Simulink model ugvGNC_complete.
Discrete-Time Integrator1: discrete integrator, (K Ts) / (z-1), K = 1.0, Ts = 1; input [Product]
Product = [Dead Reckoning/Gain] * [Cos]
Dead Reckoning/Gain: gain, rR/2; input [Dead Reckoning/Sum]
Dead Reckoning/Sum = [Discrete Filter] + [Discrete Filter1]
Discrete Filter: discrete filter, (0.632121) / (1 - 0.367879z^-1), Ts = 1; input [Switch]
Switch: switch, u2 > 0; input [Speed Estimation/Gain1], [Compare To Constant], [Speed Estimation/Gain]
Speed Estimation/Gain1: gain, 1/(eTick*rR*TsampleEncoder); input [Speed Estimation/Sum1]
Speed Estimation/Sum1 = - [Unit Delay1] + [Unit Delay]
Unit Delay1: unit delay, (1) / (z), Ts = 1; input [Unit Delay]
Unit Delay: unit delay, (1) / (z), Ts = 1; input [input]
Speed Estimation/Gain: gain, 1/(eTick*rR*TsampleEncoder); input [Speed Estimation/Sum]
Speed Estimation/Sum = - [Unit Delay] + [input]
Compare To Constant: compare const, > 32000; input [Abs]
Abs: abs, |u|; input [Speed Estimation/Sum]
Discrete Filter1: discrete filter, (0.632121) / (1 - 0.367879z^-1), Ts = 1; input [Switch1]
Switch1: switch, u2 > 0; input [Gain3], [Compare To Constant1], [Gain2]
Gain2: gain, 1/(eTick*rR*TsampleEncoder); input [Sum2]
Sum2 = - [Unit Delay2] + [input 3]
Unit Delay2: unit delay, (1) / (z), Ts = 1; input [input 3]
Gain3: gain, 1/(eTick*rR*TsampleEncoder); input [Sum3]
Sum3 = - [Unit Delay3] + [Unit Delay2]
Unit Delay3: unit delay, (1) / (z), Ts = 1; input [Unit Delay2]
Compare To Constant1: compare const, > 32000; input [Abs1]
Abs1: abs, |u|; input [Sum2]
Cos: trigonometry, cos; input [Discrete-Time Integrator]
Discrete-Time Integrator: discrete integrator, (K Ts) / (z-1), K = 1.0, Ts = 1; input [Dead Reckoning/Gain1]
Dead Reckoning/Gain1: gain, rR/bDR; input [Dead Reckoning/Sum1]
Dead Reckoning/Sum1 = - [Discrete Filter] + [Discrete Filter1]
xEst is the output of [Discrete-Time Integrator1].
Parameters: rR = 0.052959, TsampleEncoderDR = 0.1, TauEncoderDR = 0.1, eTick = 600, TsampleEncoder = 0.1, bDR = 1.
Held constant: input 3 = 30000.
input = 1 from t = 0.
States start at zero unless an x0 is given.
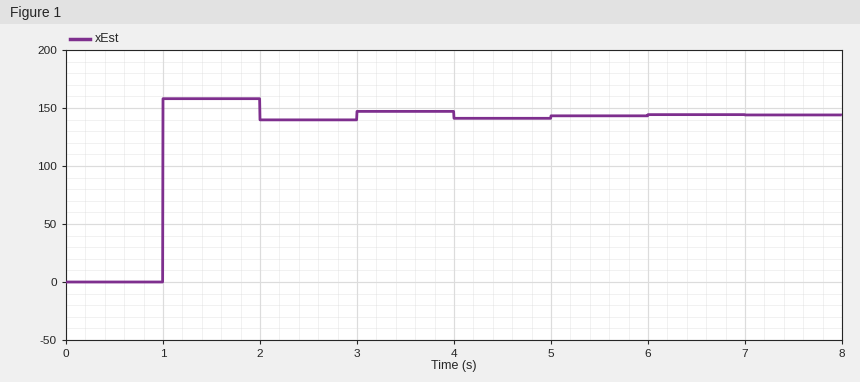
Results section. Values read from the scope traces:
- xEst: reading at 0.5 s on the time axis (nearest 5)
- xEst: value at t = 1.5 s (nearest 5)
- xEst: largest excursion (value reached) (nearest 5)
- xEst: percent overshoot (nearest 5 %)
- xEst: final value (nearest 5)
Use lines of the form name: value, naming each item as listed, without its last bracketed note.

xEst: reading at 0.5 s on the time axis: 0
xEst: value at t = 1.5 s: 160
xEst: largest excursion (value reached): 160
xEst: percent overshoot: 10 %
xEst: final value: 145
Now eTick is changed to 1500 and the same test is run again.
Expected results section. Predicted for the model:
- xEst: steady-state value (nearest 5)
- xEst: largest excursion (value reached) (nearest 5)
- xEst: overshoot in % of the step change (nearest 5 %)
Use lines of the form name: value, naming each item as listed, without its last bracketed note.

xEst: steady-state value: 70
xEst: largest excursion (value reached): 80
xEst: overshoot in % of the step change: 10 %
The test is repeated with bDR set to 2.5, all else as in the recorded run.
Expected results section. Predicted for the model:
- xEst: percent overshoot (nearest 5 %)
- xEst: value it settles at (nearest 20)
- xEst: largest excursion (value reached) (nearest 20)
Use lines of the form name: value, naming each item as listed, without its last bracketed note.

xEst: percent overshoot: 10 %
xEst: value it settles at: 180
xEst: largest excursion (value reached): 200
